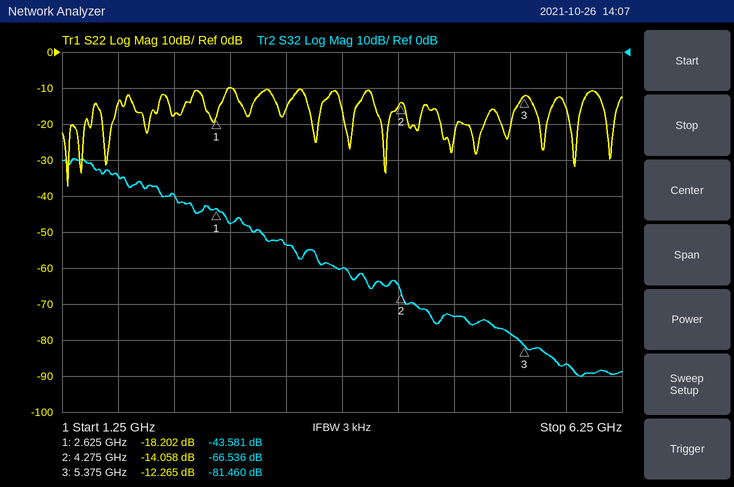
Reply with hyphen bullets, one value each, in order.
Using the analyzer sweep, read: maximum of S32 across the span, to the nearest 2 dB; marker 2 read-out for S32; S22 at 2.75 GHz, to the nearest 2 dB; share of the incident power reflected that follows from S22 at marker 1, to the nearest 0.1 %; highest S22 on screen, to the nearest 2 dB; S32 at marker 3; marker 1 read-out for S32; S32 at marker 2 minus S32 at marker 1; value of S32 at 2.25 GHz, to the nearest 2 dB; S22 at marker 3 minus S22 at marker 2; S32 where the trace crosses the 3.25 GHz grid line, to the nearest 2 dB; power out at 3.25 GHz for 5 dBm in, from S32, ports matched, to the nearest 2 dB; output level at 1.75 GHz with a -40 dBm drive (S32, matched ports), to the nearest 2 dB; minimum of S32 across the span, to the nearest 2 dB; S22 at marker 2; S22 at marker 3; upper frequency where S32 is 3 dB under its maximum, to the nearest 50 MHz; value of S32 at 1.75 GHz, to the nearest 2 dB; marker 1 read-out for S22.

- -30 dB
- -66.536 dB
- -10 dB
- 1.5 %
- -10 dB
- -81.460 dB
- -43.581 dB
- -22.955 dB
- -40 dB
- 1.793 dB
- -54 dB
- -48 dBm
- -74 dBm
- -90 dB
- -14.058 dB
- -12.265 dB
- 1.55 GHz
- -34 dB
- -18.202 dB
